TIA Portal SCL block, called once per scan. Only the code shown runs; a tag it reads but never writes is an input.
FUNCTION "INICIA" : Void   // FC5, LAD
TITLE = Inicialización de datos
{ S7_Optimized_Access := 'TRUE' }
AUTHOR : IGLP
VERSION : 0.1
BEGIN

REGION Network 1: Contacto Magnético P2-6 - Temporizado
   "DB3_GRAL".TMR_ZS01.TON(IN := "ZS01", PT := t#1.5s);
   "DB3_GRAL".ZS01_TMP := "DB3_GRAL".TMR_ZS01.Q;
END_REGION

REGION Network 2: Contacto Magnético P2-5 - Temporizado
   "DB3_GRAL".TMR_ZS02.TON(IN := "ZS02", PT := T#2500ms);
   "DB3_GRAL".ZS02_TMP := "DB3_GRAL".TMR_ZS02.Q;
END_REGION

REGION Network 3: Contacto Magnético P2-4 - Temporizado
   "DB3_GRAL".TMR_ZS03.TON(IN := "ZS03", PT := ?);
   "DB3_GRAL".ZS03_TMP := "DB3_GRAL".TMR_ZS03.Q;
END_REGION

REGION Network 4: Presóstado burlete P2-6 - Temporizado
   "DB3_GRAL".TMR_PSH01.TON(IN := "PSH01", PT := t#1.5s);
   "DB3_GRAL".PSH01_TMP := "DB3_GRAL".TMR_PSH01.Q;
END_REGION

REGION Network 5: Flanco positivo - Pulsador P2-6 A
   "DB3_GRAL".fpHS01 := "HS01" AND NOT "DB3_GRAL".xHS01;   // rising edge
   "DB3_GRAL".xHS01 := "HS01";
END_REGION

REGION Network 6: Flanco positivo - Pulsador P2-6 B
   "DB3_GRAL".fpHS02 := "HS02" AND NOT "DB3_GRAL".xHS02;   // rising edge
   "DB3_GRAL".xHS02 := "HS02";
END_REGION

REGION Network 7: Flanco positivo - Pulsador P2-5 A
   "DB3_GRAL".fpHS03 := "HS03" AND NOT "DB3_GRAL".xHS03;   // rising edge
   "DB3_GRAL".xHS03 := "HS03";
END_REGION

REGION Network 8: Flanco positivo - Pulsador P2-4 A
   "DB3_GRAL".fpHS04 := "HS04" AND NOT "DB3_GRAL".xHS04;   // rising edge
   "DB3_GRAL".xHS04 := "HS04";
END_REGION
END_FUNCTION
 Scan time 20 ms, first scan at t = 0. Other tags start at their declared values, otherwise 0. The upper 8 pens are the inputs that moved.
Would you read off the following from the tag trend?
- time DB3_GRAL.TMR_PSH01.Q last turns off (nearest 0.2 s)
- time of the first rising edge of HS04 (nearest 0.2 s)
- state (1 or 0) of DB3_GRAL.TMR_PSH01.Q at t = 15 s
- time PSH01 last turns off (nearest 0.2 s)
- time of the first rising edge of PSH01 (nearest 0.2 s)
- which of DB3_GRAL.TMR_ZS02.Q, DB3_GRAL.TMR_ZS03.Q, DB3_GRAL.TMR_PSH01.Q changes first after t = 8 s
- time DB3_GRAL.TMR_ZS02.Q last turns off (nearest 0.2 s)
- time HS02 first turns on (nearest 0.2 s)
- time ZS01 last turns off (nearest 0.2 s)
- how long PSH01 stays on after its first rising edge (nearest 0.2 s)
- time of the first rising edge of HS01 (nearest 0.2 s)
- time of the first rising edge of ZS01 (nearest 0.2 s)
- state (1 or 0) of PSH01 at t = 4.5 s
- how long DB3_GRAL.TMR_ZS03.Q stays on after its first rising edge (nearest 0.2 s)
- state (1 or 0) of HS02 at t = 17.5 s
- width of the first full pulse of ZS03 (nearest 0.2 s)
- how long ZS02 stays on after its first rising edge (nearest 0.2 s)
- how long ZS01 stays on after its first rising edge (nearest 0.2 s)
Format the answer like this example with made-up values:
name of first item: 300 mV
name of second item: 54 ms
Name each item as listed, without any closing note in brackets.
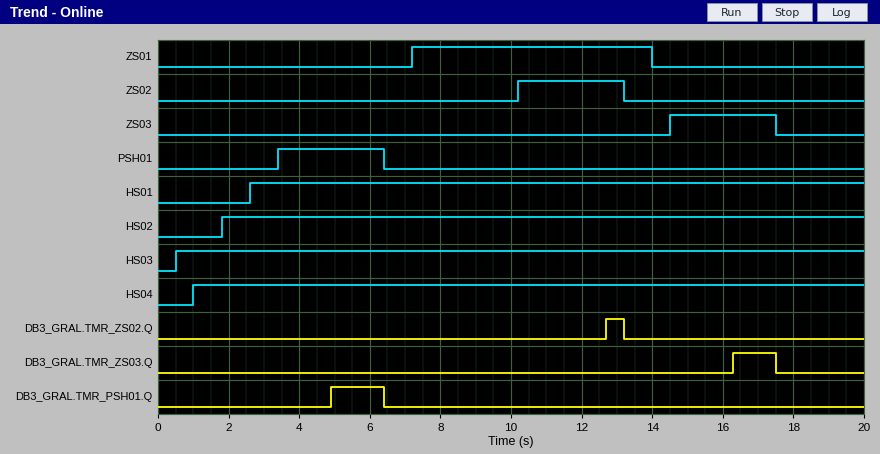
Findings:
time DB3_GRAL.TMR_PSH01.Q last turns off: 6.4 s
time of the first rising edge of HS04: 1.0 s
state (1 or 0) of DB3_GRAL.TMR_PSH01.Q at t = 15 s: 0
time PSH01 last turns off: 6.4 s
time of the first rising edge of PSH01: 3.4 s
which of DB3_GRAL.TMR_ZS02.Q, DB3_GRAL.TMR_ZS03.Q, DB3_GRAL.TMR_PSH01.Q changes first after t = 8 s: DB3_GRAL.TMR_ZS02.Q
time DB3_GRAL.TMR_ZS02.Q last turns off: 13.2 s
time HS02 first turns on: 1.8 s
time ZS01 last turns off: 14.0 s
how long PSH01 stays on after its first rising edge: 3.0 s
time of the first rising edge of HS01: 2.6 s
time of the first rising edge of ZS01: 7.2 s
state (1 or 0) of PSH01 at t = 4.5 s: 1
how long DB3_GRAL.TMR_ZS03.Q stays on after its first rising edge: 1.2 s
state (1 or 0) of HS02 at t = 17.5 s: 1
width of the first full pulse of ZS03: 3.0 s
how long ZS02 stays on after its first rising edge: 3.0 s
how long ZS01 stays on after its first rising edge: 6.8 s
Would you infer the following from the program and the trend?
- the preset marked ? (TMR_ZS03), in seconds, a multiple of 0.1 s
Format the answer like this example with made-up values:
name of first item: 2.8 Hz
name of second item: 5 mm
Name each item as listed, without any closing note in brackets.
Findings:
the preset marked ? (TMR_ZS03), in seconds, a multiple of 0.1 s: 1.8 s
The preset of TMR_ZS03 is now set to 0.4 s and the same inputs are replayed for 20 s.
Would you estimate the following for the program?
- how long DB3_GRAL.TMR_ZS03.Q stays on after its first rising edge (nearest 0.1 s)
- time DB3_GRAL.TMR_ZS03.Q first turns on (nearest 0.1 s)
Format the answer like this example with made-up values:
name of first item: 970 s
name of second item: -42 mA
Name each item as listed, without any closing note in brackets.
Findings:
how long DB3_GRAL.TMR_ZS03.Q stays on after its first rising edge: 2.6 s
time DB3_GRAL.TMR_ZS03.Q first turns on: 14.9 s
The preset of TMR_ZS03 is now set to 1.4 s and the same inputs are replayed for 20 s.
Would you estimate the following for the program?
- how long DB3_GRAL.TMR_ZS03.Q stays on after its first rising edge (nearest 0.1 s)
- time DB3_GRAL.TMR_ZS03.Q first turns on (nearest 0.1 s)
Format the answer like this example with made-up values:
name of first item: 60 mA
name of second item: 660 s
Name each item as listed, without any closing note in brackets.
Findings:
how long DB3_GRAL.TMR_ZS03.Q stays on after its first rising edge: 1.6 s
time DB3_GRAL.TMR_ZS03.Q first turns on: 15.9 s
